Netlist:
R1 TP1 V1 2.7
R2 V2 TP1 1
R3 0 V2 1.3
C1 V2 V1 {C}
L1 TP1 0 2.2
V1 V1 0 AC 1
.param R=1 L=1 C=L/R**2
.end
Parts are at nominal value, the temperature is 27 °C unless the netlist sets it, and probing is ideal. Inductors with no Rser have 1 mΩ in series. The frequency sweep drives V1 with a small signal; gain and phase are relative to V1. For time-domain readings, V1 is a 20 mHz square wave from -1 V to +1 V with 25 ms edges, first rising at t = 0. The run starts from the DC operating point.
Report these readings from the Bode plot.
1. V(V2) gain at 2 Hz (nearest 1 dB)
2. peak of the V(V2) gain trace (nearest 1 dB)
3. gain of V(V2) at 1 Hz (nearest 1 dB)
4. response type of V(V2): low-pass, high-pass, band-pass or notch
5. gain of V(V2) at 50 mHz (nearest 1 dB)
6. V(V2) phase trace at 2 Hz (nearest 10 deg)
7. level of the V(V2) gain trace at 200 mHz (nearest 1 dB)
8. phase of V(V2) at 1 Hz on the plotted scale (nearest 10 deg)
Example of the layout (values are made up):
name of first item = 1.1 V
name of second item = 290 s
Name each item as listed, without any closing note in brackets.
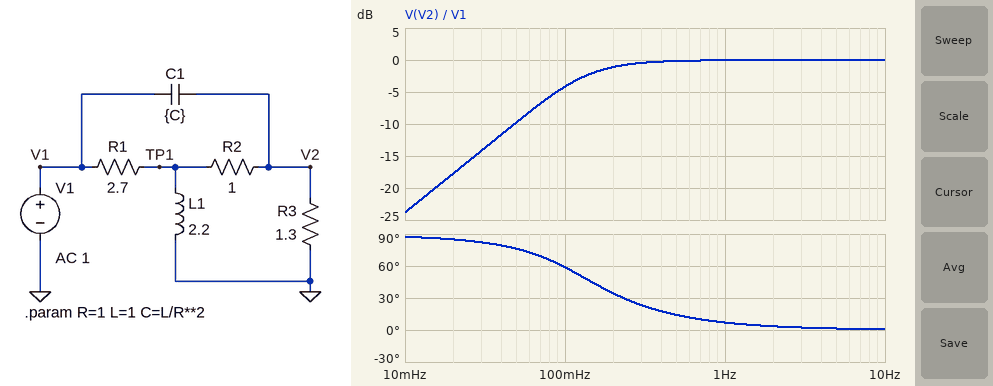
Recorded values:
V(V2) gain at 2 Hz = 0 dB
peak of the V(V2) gain trace = 0 dB
gain of V(V2) at 1 Hz = 0 dB
response type of V(V2): low-pass, high-pass, band-pass or notch = high-pass
gain of V(V2) at 50 mHz = -10 dB
V(V2) phase trace at 2 Hz = 0 deg
level of the V(V2) gain trace at 200 mHz = -1 dB
phase of V(V2) at 1 Hz on the plotted scale = 10 deg
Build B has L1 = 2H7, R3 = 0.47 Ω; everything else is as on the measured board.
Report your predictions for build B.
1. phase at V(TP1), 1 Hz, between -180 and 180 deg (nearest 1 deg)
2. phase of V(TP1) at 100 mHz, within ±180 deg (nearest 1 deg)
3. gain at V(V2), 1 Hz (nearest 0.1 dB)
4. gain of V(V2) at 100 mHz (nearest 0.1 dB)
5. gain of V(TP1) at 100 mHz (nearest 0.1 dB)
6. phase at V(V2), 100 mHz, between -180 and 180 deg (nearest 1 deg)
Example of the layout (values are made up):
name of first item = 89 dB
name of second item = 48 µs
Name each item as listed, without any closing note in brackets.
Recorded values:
phase at V(TP1), 1 Hz, between -180 and 180 deg = 16 deg
phase of V(TP1) at 100 mHz, within ±180 deg = 52 deg
gain at V(V2), 1 Hz = -0.5 dB
gain of V(V2) at 100 mHz = -10.5 dB
gain of V(TP1) at 100 mHz = -8.4 dB
phase at V(V2), 100 mHz, between -180 and 180 deg = 64 deg
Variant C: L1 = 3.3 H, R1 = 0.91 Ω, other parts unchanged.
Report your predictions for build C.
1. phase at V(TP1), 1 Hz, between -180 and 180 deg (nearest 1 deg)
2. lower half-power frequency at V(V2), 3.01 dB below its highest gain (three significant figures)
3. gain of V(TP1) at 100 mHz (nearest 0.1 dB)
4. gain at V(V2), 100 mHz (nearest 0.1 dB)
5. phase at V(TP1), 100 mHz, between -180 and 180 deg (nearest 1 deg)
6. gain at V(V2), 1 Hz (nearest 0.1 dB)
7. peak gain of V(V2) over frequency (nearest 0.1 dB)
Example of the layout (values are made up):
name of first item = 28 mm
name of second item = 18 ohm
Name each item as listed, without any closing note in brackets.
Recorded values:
phase at V(TP1), 1 Hz, between -180 and 180 deg = 5 deg
lower half-power frequency at V(V2), 3.01 dB below its highest gain = 138 mHz
gain of V(TP1) at 100 mHz = -2.3 dB
gain at V(V2), 100 mHz = -4.0 dB
phase at V(TP1), 100 mHz, between -180 and 180 deg = 25 deg
gain at V(V2), 1 Hz = -0.1 dB
peak gain of V(V2) over frequency = 0 dB
